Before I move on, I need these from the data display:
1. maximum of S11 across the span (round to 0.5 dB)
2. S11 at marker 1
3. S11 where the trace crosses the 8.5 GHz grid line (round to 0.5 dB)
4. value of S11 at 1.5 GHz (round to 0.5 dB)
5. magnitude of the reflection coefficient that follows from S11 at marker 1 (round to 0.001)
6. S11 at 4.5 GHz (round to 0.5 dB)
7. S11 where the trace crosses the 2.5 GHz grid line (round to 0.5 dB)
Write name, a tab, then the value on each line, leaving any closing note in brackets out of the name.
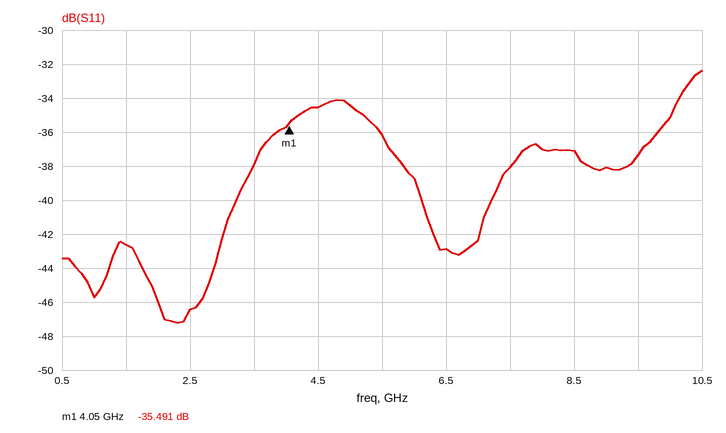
maximum of S11 across the span	-32.5 dB
S11 at marker 1	-35.491 dB
S11 where the trace crosses the 8.5 GHz grid line	-37.0 dB
value of S11 at 1.5 GHz	-42.5 dB
magnitude of the reflection coefficient that follows from S11 at marker 1	0.017
S11 at 4.5 GHz	-34.5 dB
S11 where the trace crosses the 2.5 GHz grid line	-46.5 dB
